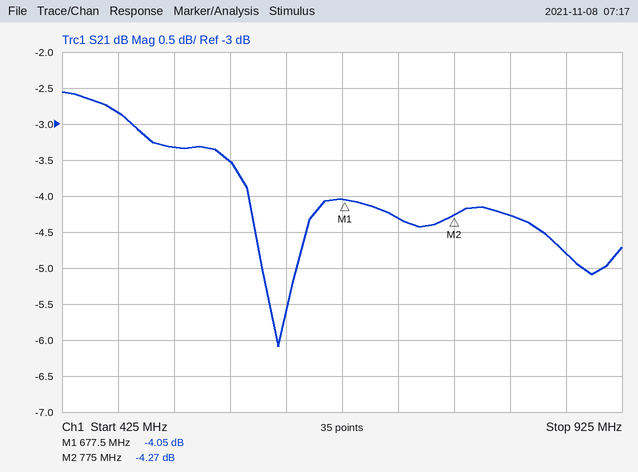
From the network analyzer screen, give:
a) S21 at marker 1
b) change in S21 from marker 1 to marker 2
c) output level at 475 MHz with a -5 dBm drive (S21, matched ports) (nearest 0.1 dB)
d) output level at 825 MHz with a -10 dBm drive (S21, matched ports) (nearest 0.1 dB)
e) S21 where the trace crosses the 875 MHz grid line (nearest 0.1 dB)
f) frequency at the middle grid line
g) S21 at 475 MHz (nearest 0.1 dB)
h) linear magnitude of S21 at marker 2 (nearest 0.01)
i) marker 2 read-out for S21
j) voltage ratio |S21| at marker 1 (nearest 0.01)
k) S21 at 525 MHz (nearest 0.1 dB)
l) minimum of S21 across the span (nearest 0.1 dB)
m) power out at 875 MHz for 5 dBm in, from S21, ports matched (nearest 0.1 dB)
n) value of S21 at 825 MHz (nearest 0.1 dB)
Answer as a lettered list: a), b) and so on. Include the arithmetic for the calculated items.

a) -4.05 dB
b) -4.27 − (-4.05) = -0.22 dB
c) -5 dBm + (-2.8 dB) = -7.8 dBm
d) -10 dBm + (-4.3 dB) = -14.3 dBm
e) -4.8 dB
f) 675 MHz
g) -2.8 dB
h) 10^(-4.27/20) ≈ 0.61
i) -4.27 dB
j) 10^(-4.05/20) ≈ 0.63
k) -3.3 dB
l) -6.1 dB
m) 5 dBm + (-4.8 dB) = 0.2 dBm
n) -4.3 dB
